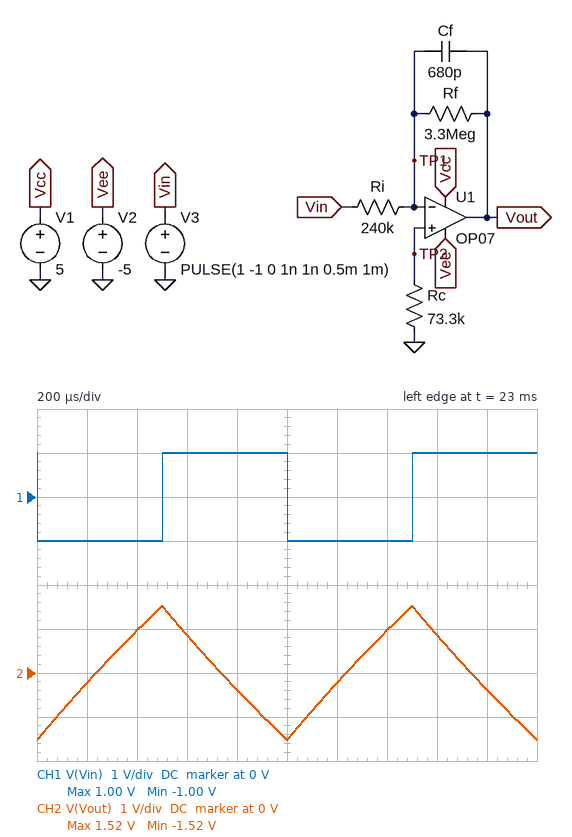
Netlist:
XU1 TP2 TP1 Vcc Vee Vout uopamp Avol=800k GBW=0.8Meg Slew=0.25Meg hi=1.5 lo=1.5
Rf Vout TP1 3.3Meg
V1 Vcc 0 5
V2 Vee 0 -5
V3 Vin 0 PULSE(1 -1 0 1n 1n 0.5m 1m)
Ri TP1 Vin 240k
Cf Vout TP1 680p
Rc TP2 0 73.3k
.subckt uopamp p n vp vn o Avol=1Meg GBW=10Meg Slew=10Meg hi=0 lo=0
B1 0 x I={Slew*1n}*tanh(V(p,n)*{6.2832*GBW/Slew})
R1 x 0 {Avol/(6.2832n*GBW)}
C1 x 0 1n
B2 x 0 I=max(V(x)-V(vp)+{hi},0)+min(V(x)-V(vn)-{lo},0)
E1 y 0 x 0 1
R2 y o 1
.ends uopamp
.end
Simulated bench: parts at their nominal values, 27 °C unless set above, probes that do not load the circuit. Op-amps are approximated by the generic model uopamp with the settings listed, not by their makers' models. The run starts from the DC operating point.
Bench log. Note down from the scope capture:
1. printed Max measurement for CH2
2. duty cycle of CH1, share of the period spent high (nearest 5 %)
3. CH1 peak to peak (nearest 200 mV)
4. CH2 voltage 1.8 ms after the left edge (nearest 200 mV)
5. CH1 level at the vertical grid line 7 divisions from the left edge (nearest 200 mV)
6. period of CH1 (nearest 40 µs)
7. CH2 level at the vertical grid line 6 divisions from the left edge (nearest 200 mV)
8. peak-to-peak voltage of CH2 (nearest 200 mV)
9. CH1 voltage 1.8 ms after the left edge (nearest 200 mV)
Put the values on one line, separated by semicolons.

1.52 V; 50 %; 2.0 V; -400 mV; -1.0 V; 1.00 ms; -200 mV; 3.0 V; 1.0 V
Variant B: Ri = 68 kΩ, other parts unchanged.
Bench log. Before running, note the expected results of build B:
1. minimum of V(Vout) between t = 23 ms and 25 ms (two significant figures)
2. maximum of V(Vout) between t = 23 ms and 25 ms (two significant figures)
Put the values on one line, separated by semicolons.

-3.5 V; 3.5 V
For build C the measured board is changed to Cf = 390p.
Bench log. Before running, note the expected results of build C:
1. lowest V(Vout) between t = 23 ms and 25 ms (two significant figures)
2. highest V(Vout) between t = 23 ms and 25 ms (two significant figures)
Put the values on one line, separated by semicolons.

-2.6 V; 2.6 V
